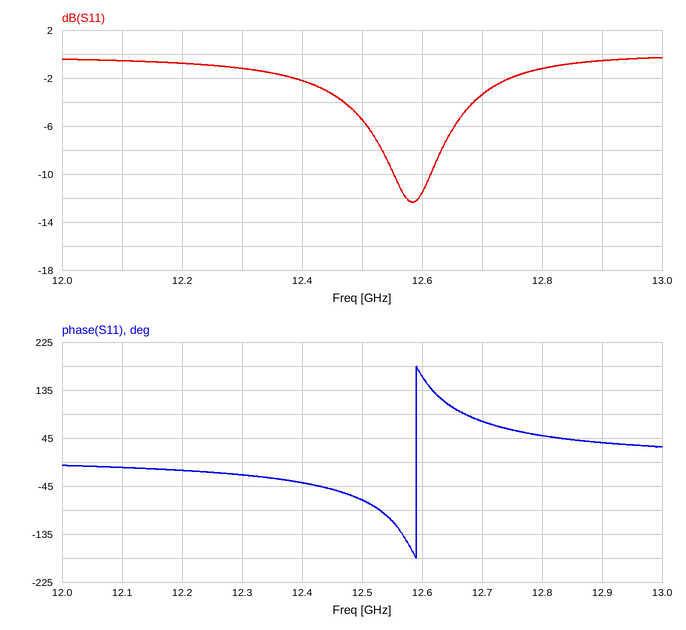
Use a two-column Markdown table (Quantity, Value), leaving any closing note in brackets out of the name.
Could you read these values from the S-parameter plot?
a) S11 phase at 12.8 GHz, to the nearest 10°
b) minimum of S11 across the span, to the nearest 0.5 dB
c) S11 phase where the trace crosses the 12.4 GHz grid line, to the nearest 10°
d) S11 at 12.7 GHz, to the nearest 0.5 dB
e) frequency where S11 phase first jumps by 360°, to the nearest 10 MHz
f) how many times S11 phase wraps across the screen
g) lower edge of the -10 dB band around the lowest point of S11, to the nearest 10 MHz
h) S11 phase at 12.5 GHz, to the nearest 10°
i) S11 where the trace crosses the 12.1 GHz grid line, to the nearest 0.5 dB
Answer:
| Quantity | Value |
|---|---|
| S11 phase at 12.8 GHz, to the nearest 10° | 50° |
| minimum of S11 across the span, to the nearest 0.5 dB | -12.5 dB |
| S11 phase where the trace crosses the 12.4 GHz grid line, to the nearest 10° | -40° |
| S11 at 12.7 GHz, to the nearest 0.5 dB | -3.5 dB |
| frequency where S11 phase first jumps by 360°, to the nearest 10 MHz | 12.59 GHz |
| how many times S11 phase wraps across the screen | 1 |
| lower edge of the -10 dB band around the lowest point of S11, to the nearest 10 MHz | 12.55 GHz |
| S11 phase at 12.5 GHz, to the nearest 10° | -70° |
| S11 where the trace crosses the 12.1 GHz grid line, to the nearest 0.5 dB | -0.5 dB |
